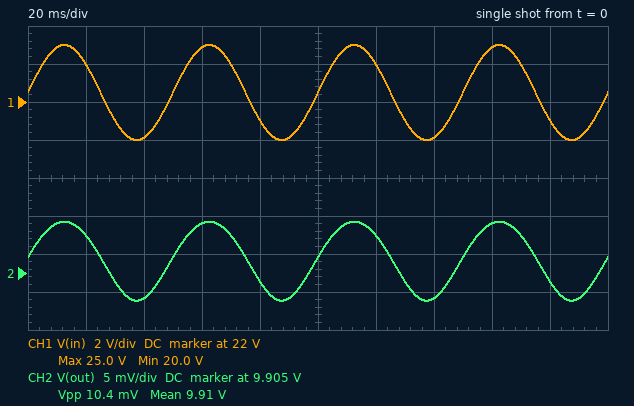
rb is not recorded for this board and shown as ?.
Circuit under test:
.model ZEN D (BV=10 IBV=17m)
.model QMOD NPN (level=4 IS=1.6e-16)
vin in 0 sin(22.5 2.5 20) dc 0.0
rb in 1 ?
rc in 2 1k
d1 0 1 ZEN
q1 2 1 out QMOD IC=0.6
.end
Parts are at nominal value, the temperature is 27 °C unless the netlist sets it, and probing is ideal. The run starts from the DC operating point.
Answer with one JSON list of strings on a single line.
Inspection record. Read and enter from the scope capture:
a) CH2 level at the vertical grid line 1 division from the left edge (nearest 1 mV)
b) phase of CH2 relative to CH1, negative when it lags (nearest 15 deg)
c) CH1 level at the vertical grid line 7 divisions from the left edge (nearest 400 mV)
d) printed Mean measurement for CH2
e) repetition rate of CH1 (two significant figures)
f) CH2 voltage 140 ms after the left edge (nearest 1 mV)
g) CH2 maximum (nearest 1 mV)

["9.910 V", "0 deg", "20.0 V", "9.91 V", "20 Hz", "9.902 V", "9.912 V"]
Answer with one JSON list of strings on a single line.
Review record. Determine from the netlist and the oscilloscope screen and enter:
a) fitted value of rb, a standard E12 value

["27 kΩ"]
